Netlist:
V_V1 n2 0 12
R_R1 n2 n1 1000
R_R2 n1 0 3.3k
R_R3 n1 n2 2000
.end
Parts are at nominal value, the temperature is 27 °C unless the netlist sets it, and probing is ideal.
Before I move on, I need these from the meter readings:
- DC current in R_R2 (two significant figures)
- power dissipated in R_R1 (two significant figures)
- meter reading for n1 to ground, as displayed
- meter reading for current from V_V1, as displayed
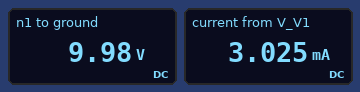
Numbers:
3.0 mA
4.1 mW
9.98 V
3.025 mA
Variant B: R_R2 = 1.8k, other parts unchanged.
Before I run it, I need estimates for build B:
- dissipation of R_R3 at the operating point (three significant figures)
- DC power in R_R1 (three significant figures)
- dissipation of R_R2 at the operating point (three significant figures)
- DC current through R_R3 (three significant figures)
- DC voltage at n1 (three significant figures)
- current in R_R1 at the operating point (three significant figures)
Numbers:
5.26 mW
10.5 mW
42.6 mW
1.62 mA
8.76 V
3.24 mA
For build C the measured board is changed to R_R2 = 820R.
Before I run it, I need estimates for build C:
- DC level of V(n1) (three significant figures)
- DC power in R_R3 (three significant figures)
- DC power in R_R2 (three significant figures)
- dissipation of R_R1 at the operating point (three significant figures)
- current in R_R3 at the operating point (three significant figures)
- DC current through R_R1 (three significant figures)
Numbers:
6.62 V
14.5 mW
53.4 mW
29.0 mW
2.69 mA
5.38 mA
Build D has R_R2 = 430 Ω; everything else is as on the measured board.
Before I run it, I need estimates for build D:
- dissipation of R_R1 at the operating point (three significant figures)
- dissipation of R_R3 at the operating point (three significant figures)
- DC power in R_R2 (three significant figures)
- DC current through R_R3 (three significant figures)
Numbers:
53.2 mW
26.6 mW
51.5 mW
3.65 mA
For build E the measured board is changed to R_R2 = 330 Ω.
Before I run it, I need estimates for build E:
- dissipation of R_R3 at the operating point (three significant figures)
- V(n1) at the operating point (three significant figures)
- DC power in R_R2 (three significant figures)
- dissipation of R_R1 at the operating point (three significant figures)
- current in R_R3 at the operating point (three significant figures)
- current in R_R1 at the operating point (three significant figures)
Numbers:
32.2 mW
3.97 V
47.8 mW
64.4 mW
4.01 mA
8.03 mA
